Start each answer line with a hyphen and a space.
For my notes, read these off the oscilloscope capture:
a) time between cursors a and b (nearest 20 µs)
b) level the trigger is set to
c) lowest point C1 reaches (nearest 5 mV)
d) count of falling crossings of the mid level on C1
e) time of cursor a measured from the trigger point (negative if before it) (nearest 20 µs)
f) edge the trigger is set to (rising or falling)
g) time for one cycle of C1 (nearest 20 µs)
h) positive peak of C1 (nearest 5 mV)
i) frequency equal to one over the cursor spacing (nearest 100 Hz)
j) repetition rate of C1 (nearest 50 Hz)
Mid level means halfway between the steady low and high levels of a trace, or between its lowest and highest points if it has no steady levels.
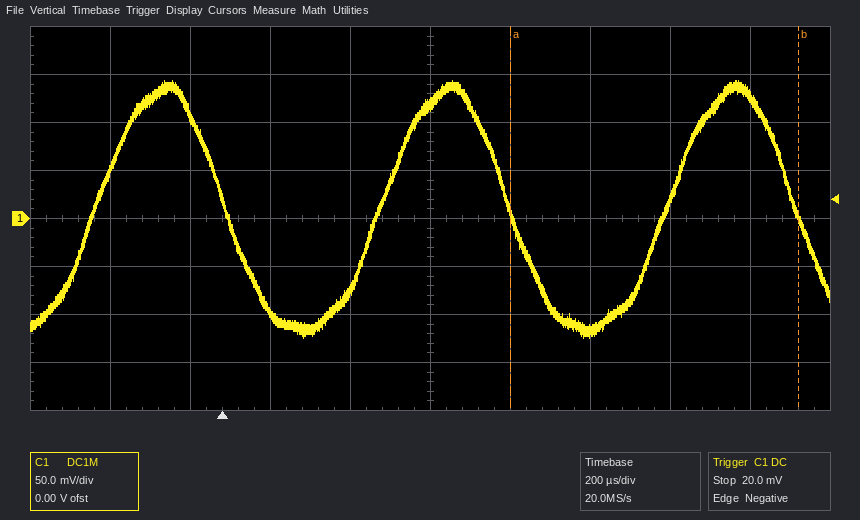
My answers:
- 720 µs
- 20.0 mV
- -125 mV
- 3
- +720 µs
- falling
- 720 µs
- 145 mV
- 1.4 kHz
- 1.40 kHz
